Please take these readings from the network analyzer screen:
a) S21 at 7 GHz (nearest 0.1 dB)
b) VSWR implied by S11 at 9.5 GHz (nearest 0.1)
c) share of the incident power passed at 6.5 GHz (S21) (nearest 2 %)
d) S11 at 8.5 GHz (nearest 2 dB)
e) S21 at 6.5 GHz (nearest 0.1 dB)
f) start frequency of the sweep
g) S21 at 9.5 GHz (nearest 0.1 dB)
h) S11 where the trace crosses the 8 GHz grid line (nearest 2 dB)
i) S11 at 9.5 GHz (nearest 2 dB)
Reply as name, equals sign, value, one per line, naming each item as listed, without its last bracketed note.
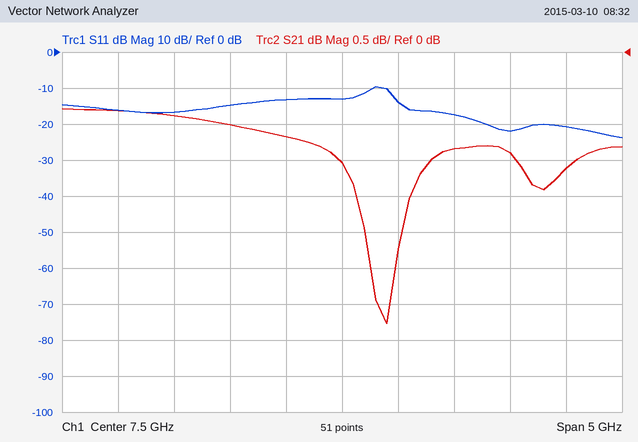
S21 at 7 GHz = -1.2 dB
VSWR implied by S11 at 9.5 GHz = 1.2
share of the incident power passed at 6.5 GHz (S21) = 80 %
S11 at 8.5 GHz = -18 dB
S21 at 6.5 GHz = -1.0 dB
start frequency of the sweep = 5 GHz
S21 at 9.5 GHz = -1.6 dB
S11 where the trace crosses the 8 GHz grid line = -14 dB
S11 at 9.5 GHz = -20 dB
